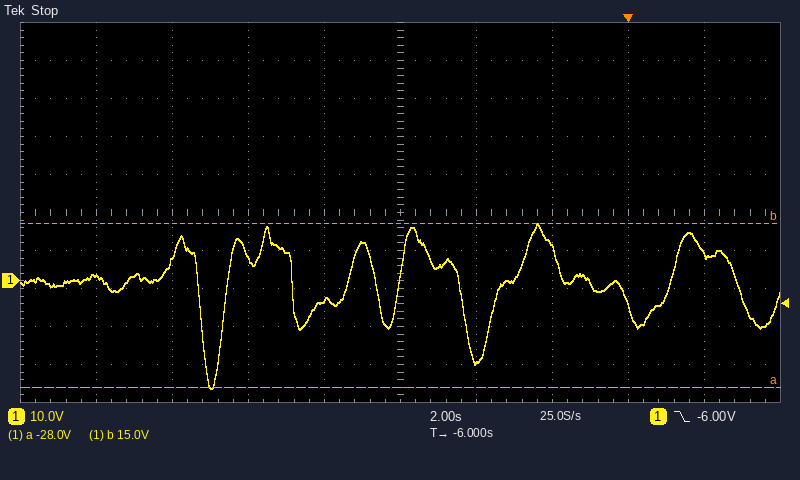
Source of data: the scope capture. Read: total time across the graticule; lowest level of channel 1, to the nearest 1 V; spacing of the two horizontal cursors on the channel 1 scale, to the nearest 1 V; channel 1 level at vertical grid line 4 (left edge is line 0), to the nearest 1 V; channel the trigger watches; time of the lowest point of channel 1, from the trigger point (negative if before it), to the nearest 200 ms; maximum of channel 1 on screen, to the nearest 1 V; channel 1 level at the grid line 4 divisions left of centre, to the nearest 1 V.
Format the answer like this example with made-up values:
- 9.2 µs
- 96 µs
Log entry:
- 20 s
- -28 V
- 43 V
- -5 V
- channel 1
- -11.0 s
- 15 V
- 1 V
